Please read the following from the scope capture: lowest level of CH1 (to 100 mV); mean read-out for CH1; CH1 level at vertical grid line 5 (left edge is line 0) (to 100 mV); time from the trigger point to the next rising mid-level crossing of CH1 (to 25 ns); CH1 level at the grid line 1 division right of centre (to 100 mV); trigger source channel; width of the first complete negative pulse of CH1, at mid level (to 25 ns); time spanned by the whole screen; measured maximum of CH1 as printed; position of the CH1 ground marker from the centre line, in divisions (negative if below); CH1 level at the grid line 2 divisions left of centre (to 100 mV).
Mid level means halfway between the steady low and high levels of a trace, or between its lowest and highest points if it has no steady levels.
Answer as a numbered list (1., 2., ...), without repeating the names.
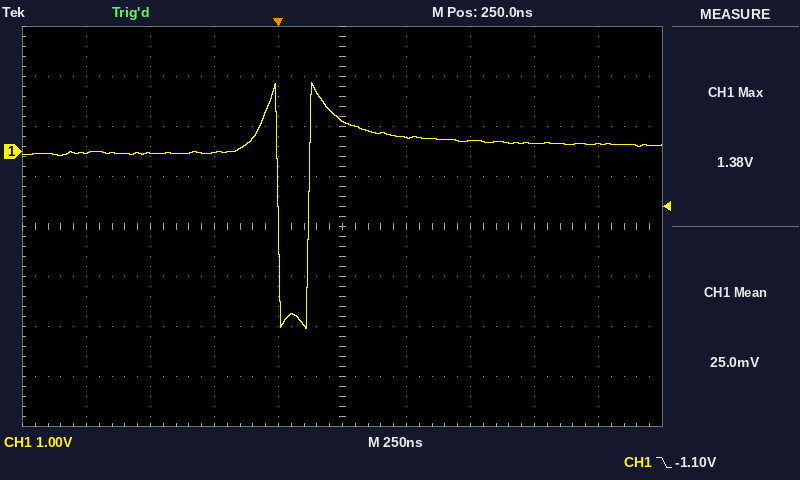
1. -3.5 V
2. 25.0 mV
3. 600 mV
4. 125 ns
5. 300 mV
6. CH1
7. 125 ns
8. 2.5 µs
9. 1.38 V
10. +1.5 div
11. 0.0 V
